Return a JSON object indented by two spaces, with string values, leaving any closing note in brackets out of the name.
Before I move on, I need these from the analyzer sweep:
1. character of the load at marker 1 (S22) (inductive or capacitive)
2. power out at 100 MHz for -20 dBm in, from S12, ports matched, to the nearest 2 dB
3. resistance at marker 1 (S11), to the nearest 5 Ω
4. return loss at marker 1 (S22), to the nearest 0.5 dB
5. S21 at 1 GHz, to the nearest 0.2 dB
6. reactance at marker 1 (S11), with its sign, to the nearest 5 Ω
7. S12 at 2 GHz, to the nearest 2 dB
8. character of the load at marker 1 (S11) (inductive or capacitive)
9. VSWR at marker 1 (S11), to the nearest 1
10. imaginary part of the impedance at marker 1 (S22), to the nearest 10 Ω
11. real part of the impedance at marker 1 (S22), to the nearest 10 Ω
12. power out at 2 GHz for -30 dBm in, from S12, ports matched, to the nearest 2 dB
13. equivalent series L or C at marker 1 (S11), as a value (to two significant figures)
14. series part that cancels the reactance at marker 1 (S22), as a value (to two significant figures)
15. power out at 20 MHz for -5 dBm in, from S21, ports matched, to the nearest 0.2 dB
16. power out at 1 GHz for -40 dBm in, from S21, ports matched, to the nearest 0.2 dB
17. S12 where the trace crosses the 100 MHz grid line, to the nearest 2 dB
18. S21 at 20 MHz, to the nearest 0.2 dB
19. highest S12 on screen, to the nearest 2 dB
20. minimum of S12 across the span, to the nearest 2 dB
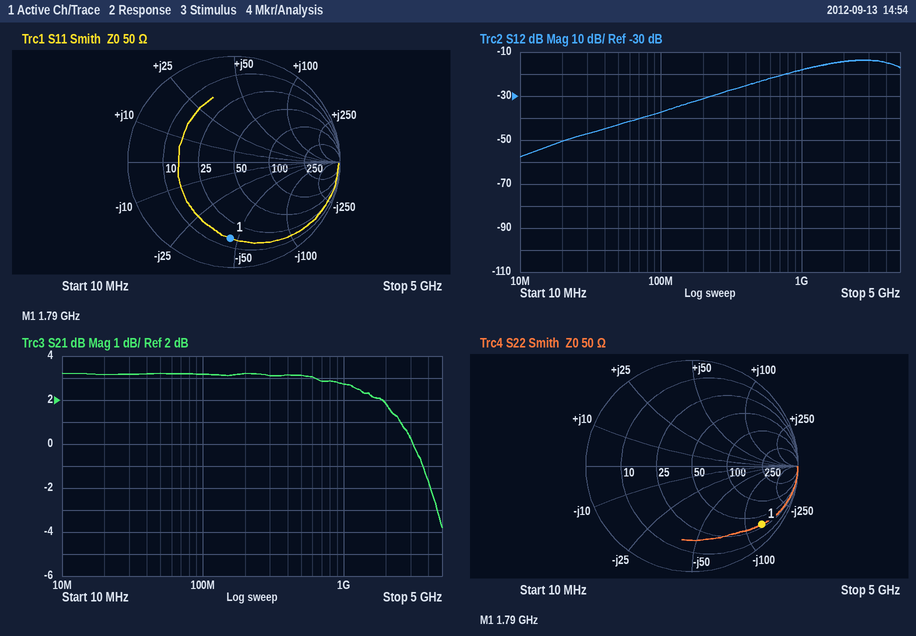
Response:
{
  "character of the load at marker 1 (S22)": "capacitive",
  "power out at 100 MHz for -20 dBm in, from S12, ports matched, to the nearest 2 dB": "-58 dBm",
  "resistance at marker 1 (S11), to the nearest 5 Ω": "15 Ω",
  "return loss at marker 1 (S22), to the nearest 0.5 dB": "1.5 dB",
  "S21 at 1 GHz, to the nearest 0.2 dB": "2.8 dB",
  "reactance at marker 1 (S11), with its sign, to the nearest 5 Ω": "-45 Ω",
  "S12 at 2 GHz, to the nearest 2 dB": "-14 dB",
  "character of the load at marker 1 (S11)": "capacitive",
  "VSWR at marker 1 (S11), to the nearest 1": "6",
  "imaginary part of the impedance at marker 1 (S22), to the nearest 10 Ω": "-130 Ω",
  "real part of the impedance at marker 1 (S22), to the nearest 10 Ω": "30 Ω",
  "power out at 2 GHz for -30 dBm in, from S12, ports matched, to the nearest 2 dB": "-44 dBm",
  "equivalent series L or C at marker 1 (S11), as a value": "2.0 pF",
  "series part that cancels the reactance at marker 1 (S22), as a value": "12 nH",
  "power out at 20 MHz for -5 dBm in, from S21, ports matched, to the nearest 0.2 dB": "-1.8 dBm",
  "power out at 1 GHz for -40 dBm in, from S21, ports matched, to the nearest 0.2 dB": "-37.2 dBm",
  "S12 where the trace crosses the 100 MHz grid line, to the nearest 2 dB": "-38 dB",
  "S21 at 20 MHz, to the nearest 0.2 dB": "3.2 dB",
  "highest S12 on screen, to the nearest 2 dB": "-14 dB",
  "minimum of S12 across the span, to the nearest 2 dB": "-58 dB"
}
